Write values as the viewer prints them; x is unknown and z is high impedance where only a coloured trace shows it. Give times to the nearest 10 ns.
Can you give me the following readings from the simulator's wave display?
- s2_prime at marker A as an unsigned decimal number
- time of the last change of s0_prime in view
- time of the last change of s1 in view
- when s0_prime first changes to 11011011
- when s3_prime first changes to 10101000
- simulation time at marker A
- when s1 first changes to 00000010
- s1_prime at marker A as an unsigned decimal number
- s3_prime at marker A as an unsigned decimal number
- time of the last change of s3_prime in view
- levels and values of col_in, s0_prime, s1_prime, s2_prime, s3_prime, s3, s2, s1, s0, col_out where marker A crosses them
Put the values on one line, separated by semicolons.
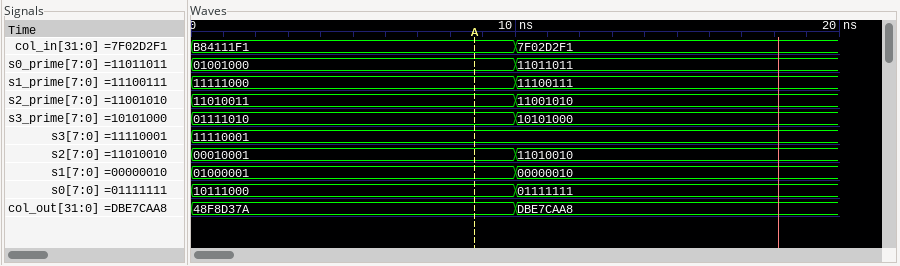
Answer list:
211; 10 ns; 10 ns; 10 ns; 10 ns; 10 ns; 10 ns; 248; 122; 10 ns; col_in=B84111F1, s0_prime=01001000, s1_prime=11111000, s2_prime=11010011, s3_prime=01111010, s3=11110001, s2=00010001, s1=01000001, s0=10111000, col_out=48F8D37A
